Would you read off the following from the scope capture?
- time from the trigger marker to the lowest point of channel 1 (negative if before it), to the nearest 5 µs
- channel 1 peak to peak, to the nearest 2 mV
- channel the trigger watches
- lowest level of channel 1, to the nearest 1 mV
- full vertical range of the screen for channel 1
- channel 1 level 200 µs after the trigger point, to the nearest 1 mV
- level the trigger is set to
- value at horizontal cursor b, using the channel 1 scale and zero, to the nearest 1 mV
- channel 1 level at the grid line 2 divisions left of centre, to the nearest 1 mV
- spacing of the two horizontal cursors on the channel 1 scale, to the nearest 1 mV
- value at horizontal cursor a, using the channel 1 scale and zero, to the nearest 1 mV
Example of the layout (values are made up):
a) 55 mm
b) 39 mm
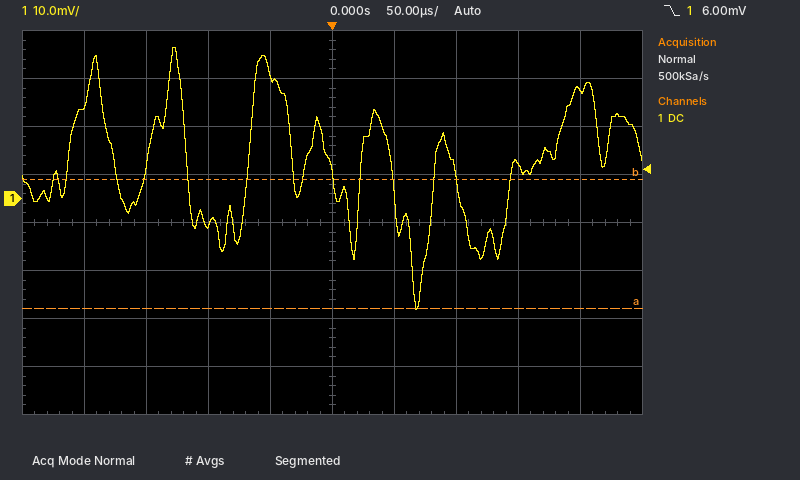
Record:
a) +70 µs
b) 54 mV
c) channel 1
d) -23 mV
e) 80 mV
f) 23 mV
g) 6.00 mV
h) 4 mV
i) -5 mV
j) 27 mV
k) -23 mV
